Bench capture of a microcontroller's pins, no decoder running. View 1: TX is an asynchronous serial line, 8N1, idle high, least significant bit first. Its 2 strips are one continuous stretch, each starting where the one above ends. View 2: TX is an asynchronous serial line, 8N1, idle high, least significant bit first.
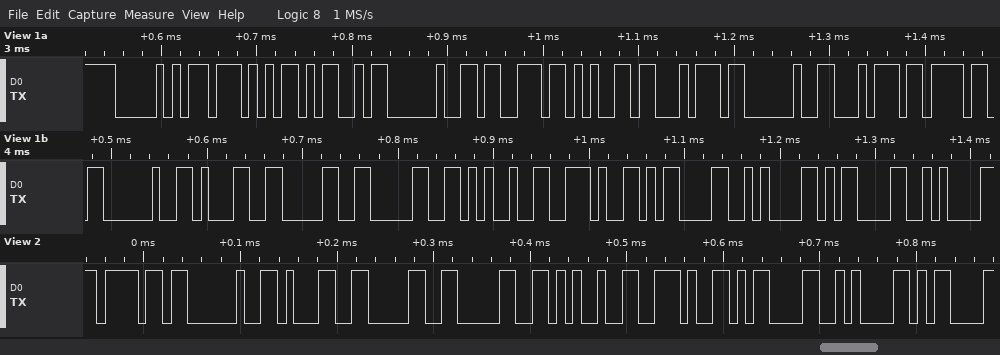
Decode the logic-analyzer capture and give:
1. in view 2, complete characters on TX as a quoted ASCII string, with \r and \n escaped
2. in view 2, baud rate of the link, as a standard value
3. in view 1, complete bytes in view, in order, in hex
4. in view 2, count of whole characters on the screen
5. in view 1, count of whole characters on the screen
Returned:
"o 100%.\r\n\r"
115200 baud
50 57 4D 20 73 65 74 20 74 6F 20 31 30 30 25 2E 0D 0A 0D 0A
10
20
